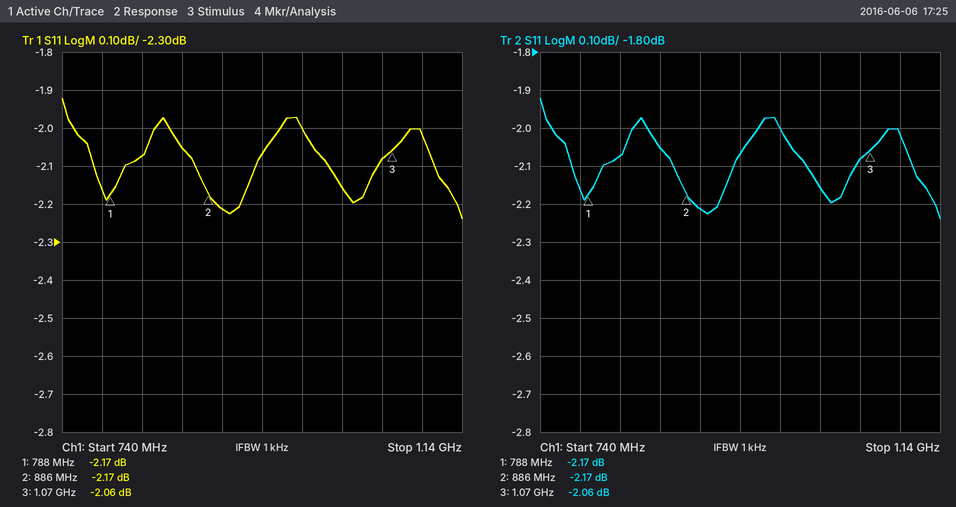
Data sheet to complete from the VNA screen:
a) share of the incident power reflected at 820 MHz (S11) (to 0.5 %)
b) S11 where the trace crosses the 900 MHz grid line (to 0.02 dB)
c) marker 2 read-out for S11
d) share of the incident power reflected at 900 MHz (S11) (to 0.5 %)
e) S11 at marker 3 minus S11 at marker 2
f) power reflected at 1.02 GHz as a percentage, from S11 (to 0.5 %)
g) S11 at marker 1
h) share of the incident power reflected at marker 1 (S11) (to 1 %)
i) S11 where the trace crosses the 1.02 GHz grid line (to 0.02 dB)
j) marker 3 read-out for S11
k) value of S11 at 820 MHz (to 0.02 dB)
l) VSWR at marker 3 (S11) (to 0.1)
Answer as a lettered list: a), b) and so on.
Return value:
a) 62.0 %
b) -2.22 dB
c) -2.17 dB
d) 60.0 %
e) 0.11 dB
f) 61.0 %
g) -2.17 dB
h) 61 %
i) -2.16 dB
j) -2.06 dB
k) -2.08 dB
l) 8.5
